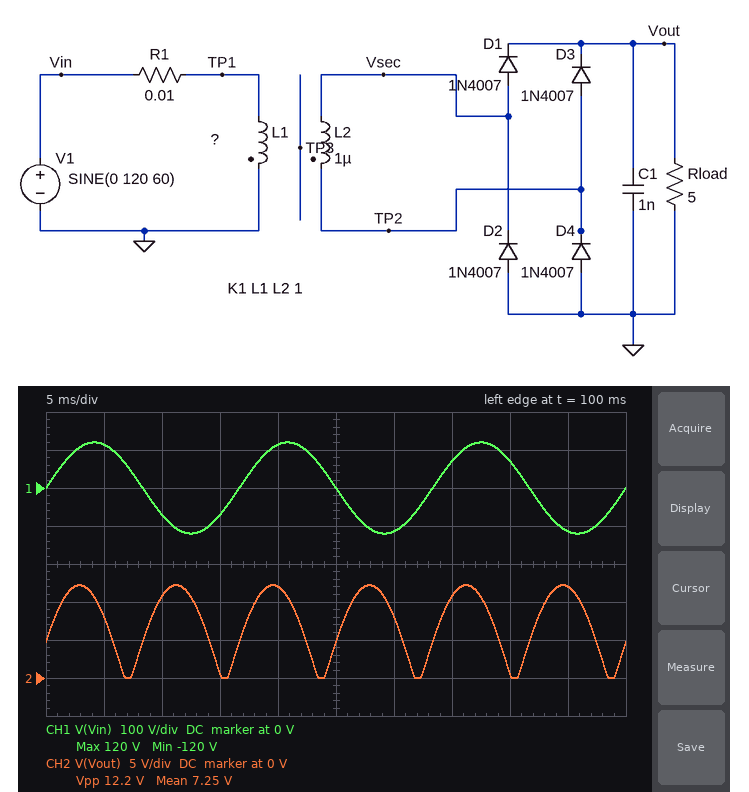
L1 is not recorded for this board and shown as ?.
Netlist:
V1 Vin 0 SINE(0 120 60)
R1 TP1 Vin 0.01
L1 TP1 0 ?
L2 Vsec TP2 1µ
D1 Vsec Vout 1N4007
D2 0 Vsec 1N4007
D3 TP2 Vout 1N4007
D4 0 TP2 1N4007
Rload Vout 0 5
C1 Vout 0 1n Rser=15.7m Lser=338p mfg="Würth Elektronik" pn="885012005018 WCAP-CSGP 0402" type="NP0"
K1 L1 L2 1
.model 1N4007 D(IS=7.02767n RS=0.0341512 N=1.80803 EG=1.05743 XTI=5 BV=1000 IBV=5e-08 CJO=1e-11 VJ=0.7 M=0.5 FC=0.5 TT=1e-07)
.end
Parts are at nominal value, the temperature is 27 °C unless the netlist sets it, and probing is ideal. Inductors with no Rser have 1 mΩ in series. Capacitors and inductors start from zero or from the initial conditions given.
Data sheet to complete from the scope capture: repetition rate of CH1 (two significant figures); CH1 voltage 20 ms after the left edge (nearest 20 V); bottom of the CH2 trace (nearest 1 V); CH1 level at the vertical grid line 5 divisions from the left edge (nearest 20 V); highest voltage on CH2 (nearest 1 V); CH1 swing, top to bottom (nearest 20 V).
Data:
60 Hz
120 V
0 V
0 V
12 V
240 V
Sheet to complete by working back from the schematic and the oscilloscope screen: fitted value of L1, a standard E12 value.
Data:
56 µH
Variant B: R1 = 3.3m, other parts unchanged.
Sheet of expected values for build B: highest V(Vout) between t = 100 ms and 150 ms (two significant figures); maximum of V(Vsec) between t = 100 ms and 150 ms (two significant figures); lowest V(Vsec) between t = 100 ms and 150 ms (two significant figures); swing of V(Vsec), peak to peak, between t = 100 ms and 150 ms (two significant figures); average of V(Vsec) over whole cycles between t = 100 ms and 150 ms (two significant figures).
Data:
14 V
15 V
-1.0 V
16 V
4.1 V
